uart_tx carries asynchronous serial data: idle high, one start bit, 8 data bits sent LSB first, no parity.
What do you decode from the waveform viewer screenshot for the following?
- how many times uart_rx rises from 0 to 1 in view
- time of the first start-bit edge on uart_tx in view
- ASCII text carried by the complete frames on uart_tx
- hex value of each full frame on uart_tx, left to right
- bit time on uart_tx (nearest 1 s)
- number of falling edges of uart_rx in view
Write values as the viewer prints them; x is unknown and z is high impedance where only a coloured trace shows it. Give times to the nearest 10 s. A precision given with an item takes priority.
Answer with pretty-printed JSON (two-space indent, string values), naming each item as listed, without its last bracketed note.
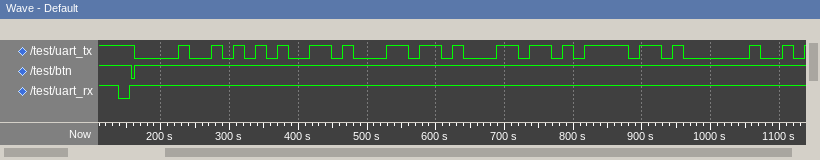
{
  "how many times uart_rx rises from 0 to 1 in view": "1",
  "time of the first start-bit edge on uart_tx in view": "160 s",
  "ASCII text carried by the complete frames on uart_tx": "\"Hello \"",
  "hex value of each full frame on uart_tx, left to right": "48, 65, 6C, 6C, 6F, 20",
  "bit time on uart_tx": "16 s",
  "number of falling edges of uart_rx in view": "1"
}
